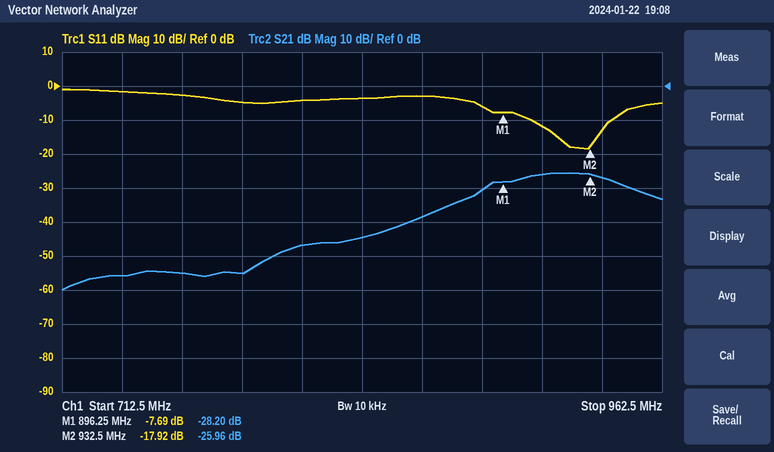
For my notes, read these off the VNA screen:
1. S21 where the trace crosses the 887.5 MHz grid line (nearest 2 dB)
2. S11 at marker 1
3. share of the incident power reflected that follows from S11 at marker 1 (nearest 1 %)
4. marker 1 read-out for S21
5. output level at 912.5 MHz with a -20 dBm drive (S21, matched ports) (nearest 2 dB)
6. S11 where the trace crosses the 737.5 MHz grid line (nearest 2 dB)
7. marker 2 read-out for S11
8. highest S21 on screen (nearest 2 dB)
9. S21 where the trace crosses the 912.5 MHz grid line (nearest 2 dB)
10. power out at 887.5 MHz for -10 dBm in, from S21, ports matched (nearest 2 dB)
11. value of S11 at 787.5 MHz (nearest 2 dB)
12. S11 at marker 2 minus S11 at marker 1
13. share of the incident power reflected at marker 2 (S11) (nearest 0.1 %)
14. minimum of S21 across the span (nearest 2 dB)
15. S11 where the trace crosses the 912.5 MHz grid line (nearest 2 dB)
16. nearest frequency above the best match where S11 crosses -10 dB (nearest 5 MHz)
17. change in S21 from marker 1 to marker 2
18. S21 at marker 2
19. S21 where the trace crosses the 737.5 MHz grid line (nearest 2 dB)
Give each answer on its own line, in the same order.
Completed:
-30 dB
-7.69 dB
17 %
-28.20 dB
-46 dBm
-2 dB
-17.92 dB
-26 dB
-26 dB
-40 dBm
-4 dB
-10.23 dB
1.6 %
-60 dB
-12 dB
940 MHz
2.24 dB
-25.96 dB
-56 dB
